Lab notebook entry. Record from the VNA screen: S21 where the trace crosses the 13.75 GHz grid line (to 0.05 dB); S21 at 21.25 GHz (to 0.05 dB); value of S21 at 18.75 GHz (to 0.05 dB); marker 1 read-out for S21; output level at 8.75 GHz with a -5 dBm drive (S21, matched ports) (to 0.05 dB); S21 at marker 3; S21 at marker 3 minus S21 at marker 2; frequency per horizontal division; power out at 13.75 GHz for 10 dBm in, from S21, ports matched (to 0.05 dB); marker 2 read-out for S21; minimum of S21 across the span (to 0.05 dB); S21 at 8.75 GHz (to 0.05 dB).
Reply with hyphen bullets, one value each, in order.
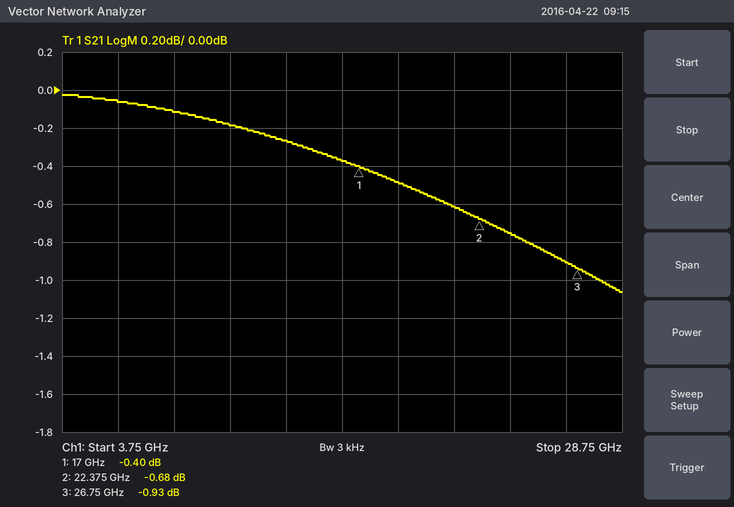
- -0.25 dB
- -0.60 dB
- -0.50 dB
- -0.40 dB
- -5.10 dBm
- -0.93 dB
- -0.25 dB
- 2.5 GHz
- 9.75 dBm
- -0.68 dB
- -1.05 dB
- -0.10 dB
